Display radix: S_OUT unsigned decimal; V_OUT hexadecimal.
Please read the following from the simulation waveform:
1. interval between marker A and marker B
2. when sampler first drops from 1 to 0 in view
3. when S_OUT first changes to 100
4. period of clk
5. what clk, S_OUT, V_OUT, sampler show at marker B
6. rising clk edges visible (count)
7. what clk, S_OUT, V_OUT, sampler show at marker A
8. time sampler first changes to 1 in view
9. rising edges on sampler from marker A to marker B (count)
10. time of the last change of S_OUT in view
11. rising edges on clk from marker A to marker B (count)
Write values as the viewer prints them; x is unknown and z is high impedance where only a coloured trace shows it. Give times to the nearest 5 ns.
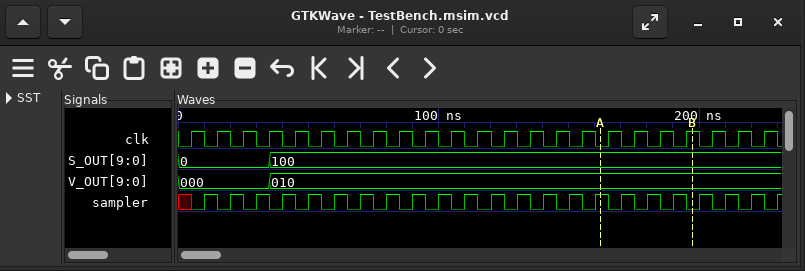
35 ns
15 ns
35 ns
10 ns
clk=1, S_OUT=100, V_OUT=010, sampler=0
23
clk=0, S_OUT=100, V_OUT=010, sampler=1
10 ns
3
35 ns
4
